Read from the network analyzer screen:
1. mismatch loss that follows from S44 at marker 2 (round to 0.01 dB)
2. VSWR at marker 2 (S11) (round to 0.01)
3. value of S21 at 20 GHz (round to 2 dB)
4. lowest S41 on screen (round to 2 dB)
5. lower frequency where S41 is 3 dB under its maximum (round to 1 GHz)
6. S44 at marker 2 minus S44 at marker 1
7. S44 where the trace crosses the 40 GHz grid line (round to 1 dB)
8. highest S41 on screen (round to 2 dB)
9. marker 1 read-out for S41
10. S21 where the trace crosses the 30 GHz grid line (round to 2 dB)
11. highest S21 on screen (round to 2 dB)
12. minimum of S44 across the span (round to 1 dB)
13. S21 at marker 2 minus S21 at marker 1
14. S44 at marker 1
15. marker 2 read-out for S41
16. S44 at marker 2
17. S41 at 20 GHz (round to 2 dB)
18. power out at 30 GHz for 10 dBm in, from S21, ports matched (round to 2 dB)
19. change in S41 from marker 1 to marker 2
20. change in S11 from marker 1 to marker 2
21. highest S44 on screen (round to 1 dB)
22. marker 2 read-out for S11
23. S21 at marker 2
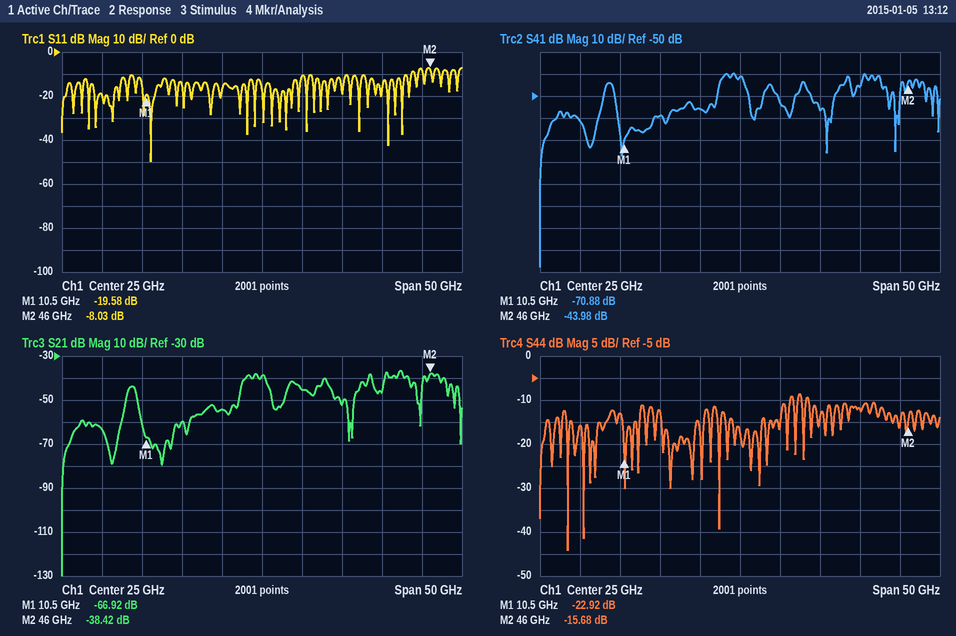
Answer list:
0.12 dB
2.32
-54 dB
-128 dB
23 GHz
7.24 dB
-12 dB
-40 dB
-70.88 dB
-46 dB
-36 dB
-44 dB
28.50 dB
-22.92 dB
-43.98 dB
-15.68 dB
-56 dB
-36 dBm
26.90 dB
11.55 dB
-9 dB
-8.03 dB
-38.42 dB
